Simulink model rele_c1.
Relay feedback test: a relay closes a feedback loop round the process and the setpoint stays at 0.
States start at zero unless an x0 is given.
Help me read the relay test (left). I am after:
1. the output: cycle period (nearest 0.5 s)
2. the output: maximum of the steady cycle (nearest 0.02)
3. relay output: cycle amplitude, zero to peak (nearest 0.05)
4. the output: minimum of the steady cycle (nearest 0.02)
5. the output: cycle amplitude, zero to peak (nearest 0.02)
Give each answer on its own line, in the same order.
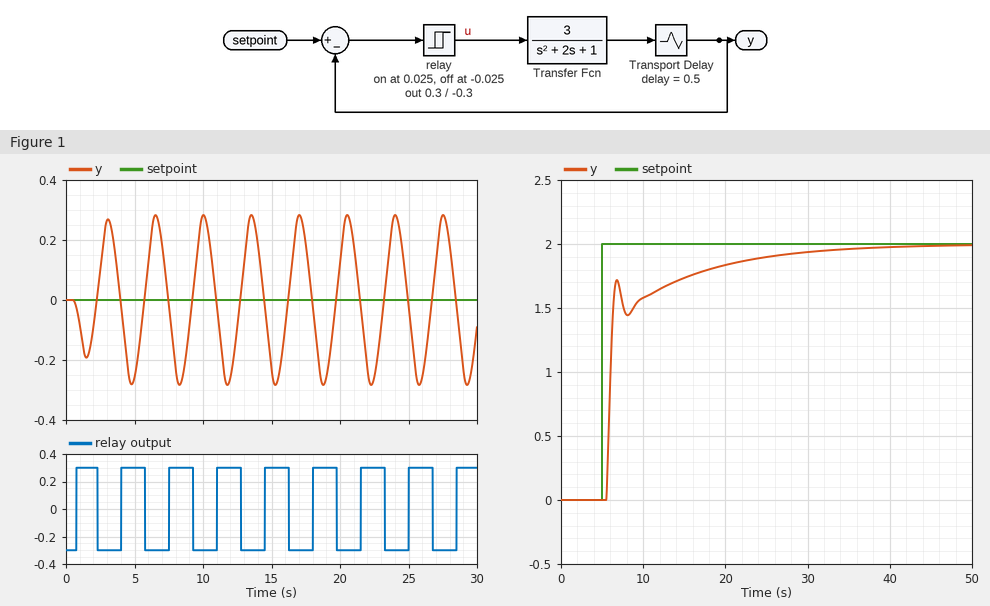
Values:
3.5 s
0.28
0.30
-0.28
0.28
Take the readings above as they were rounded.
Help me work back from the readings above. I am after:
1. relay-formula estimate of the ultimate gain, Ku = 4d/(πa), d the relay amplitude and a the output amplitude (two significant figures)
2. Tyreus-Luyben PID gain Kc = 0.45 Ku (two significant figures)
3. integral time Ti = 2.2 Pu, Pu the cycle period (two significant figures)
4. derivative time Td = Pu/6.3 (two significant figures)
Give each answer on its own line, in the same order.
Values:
1.4
0.63
7.7 s
0.56 s
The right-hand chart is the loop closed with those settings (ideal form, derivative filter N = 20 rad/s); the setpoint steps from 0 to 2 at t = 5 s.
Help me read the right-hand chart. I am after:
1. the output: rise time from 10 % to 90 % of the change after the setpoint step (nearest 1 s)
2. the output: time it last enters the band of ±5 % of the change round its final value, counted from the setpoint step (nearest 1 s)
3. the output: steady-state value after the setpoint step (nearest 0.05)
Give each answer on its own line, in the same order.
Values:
12 s
20 s
2.00
